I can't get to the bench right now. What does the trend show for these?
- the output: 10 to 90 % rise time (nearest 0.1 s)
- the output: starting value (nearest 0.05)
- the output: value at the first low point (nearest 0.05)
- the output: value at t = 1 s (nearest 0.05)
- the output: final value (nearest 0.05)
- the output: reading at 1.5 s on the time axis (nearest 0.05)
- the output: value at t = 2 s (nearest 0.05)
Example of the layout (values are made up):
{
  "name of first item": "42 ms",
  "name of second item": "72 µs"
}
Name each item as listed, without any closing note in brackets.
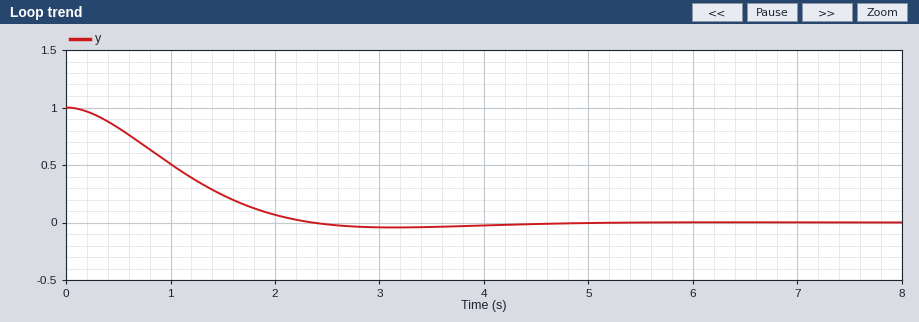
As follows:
{
  "the output: 10 to 90 % rise time": "1.5 s",
  "the output: starting value": "1.00",
  "the output: value at the first low point": "-0.05",
  "the output: value at t = 1 s": "0.50",
  "the output: final value": "0.00",
  "the output: reading at 1.5 s on the time axis": "0.25",
  "the output: value at t = 2 s": "0.05"
}
